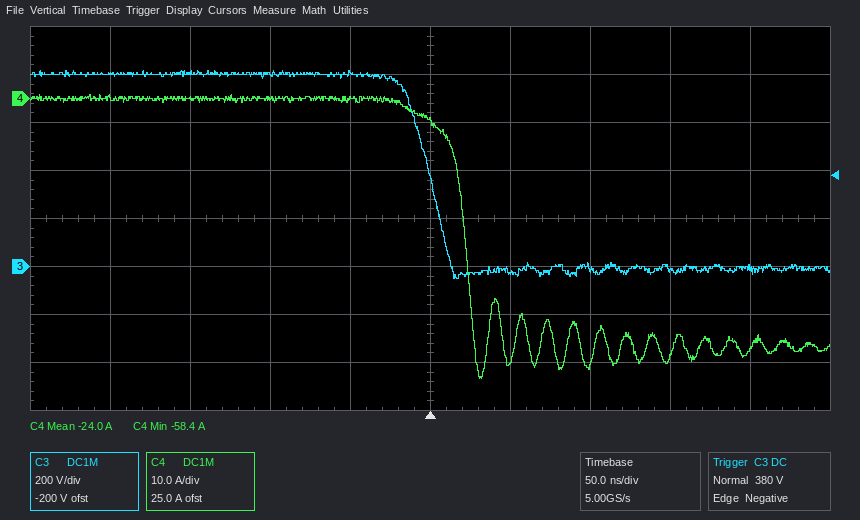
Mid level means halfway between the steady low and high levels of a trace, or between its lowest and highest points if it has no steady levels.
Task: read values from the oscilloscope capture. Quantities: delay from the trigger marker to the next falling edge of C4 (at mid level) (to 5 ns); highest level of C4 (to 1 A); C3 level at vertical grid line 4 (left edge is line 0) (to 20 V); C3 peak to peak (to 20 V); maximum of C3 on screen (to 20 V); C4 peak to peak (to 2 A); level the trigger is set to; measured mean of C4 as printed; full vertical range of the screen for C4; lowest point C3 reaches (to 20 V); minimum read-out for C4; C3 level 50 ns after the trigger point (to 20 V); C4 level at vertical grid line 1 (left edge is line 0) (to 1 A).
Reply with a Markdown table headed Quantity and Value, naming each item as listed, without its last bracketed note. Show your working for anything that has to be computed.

| Quantity | Value |
|---|---|
| delay from the trigger marker to the next falling edge of C4 (at mid level) | 20 ns |
| highest level of C4 | 1 A |
| C3 level at vertical grid line 4 (left edge is line 0) | 800 V |
| C3 peak to peak | 820 V − (-40 V) = 860 V |
| maximum of C3 on screen | 820 V |
| C4 peak to peak | 60 A |
| level the trigger is set to | 380 V |
| measured mean of C4 as printed | -24.0 A |
| full vertical range of the screen for C4 | 80 A |
| lowest point C3 reaches | -40 V |
| minimum read-out for C4 | -58.4 A |
| C3 level 50 ns after the trigger point | -20 V |
| C4 level at vertical grid line 1 (left edge is line 0) | 0 A |
